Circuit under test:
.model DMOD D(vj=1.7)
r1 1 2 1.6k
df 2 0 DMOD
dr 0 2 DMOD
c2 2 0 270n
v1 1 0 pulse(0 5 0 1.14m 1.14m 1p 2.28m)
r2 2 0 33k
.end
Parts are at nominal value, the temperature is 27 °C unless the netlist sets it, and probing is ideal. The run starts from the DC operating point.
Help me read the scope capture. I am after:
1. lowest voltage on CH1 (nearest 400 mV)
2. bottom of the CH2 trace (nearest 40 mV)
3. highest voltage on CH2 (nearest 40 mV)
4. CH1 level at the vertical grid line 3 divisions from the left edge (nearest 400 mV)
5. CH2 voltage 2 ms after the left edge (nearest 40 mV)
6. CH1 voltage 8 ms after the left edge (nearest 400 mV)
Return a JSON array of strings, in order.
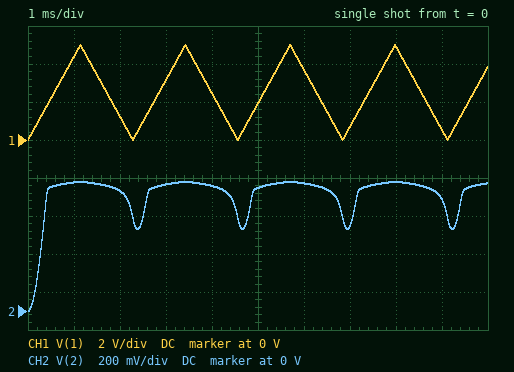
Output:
["0 V", "0 V", "680 mV", "3.2 V", "640 mV", "4.8 V"]
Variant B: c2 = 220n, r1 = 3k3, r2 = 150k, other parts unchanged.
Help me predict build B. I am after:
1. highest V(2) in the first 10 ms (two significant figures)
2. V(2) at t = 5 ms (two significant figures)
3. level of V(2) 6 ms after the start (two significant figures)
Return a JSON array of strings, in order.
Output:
["660 mV", "630 mV", "650 mV"]
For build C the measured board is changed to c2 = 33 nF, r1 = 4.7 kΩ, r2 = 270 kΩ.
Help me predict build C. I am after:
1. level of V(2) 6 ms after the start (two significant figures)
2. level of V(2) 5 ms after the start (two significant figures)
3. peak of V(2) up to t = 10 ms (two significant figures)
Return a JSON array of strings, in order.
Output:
["640 mV", "620 mV", "650 mV"]
